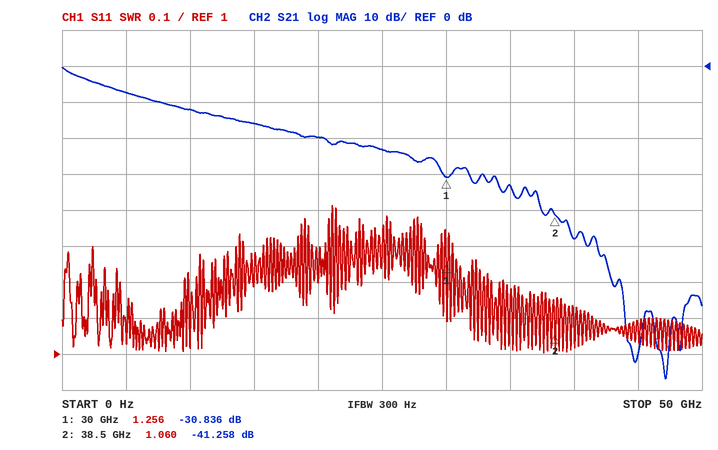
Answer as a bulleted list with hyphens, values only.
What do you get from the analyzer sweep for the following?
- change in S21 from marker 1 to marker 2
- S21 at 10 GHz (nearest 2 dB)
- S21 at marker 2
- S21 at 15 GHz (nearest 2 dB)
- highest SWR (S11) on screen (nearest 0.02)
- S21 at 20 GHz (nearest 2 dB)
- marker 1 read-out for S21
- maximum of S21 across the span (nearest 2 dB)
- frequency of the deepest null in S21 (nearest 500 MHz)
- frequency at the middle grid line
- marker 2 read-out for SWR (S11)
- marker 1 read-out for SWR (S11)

- -10.422 dB
- -12 dB
- -41.258 dB
- -16 dB
- 1.42
- -20 dB
- -30.836 dB
- 0 dB
- 47.0 GHz
- 25 GHz
- 1.060
- 1.256
